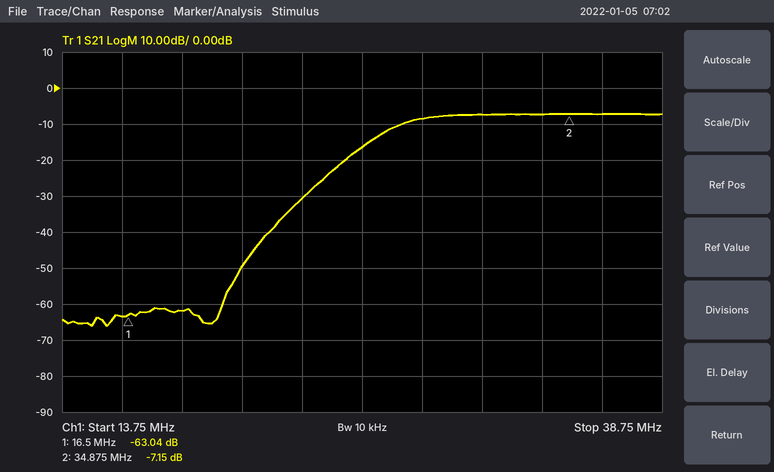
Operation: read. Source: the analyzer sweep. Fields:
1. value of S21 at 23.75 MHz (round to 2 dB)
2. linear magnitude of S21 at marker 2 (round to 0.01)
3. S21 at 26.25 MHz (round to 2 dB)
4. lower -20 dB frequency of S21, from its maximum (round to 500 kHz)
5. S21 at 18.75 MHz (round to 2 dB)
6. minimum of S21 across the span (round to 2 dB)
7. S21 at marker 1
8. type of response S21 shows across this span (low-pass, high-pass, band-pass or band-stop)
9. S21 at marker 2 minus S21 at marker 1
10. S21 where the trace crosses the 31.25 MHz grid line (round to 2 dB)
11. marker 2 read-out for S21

-30 dB
0.44
-16 dB
24.5 MHz
-62 dB
-66 dB
-63.04 dB
high-pass
55.89 dB
-8 dB
-7.15 dB
